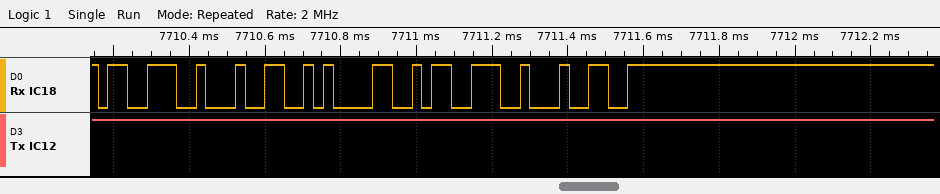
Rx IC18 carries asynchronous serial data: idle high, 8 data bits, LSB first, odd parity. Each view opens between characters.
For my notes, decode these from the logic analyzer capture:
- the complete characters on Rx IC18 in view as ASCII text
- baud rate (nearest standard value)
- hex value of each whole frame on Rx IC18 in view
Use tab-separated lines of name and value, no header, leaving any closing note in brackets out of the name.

the complete characters on Rx IC18 in view as ASCII text	"sdasd"
baud rate	38400 baud
hex value of each whole frame on Rx IC18 in view	73, 64, 61, 73, 64
